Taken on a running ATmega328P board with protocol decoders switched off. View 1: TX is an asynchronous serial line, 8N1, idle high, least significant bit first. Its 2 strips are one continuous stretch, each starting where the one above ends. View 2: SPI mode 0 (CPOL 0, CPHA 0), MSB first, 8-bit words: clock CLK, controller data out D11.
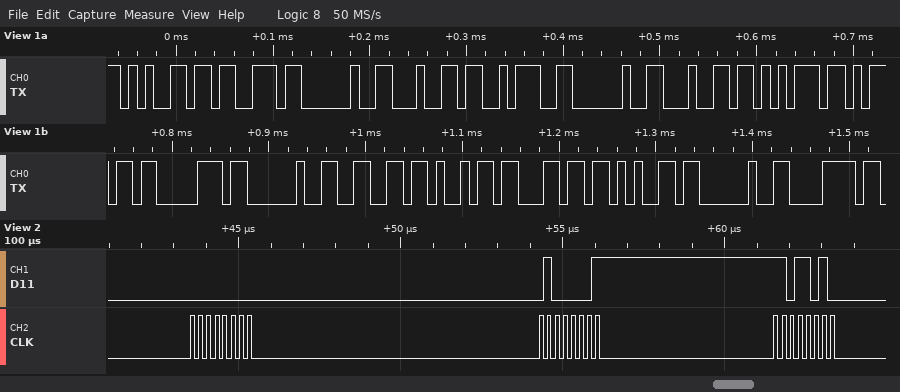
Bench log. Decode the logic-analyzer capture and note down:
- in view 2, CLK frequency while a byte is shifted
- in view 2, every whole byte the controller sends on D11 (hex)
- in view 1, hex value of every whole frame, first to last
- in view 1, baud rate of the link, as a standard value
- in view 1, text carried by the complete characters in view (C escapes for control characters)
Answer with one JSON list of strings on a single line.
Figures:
["4 MHz", "00 41 DA", "0x65 0x73 0x20 0x64 0x3A 0x20 0x64 0x75 0x6D 0x70 0x20 0x66 0x69 0x6C 0x65 0x20 0x78", "115200 baud", "\"es d: dump file x\""]
